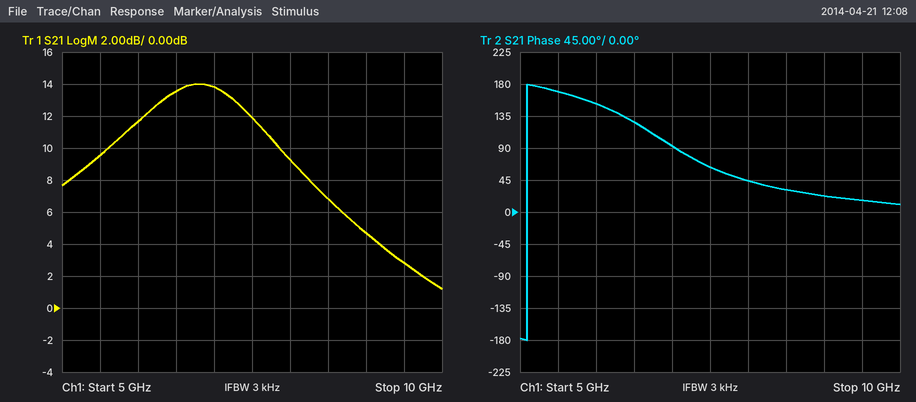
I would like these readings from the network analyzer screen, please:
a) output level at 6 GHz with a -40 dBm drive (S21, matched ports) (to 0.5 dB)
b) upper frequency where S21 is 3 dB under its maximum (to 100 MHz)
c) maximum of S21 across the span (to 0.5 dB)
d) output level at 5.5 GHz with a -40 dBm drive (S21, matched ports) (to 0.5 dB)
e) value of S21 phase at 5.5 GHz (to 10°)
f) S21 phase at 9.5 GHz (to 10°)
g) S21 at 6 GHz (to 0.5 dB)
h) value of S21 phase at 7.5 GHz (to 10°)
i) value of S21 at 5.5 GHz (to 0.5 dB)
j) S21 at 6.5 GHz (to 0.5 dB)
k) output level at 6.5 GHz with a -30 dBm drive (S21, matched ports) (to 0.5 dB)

-28.5 dBm
7.7 GHz
14.0 dB
-30.5 dBm
170°
20°
11.5 dB
60°
9.5 dB
13.5 dB
-16.5 dBm
